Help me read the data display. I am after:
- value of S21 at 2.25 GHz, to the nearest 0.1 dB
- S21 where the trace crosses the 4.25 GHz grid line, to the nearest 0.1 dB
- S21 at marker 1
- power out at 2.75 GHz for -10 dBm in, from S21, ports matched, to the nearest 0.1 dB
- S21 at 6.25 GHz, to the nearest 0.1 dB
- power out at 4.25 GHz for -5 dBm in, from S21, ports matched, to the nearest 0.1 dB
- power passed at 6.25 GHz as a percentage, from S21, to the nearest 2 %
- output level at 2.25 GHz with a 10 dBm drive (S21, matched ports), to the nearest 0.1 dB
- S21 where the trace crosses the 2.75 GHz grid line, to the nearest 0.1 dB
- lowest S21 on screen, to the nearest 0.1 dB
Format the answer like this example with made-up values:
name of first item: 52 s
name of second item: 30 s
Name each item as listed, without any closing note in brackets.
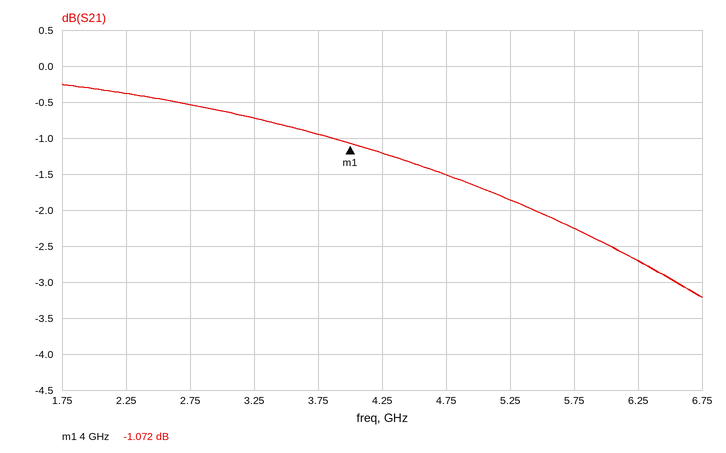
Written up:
value of S21 at 2.25 GHz, to the nearest 0.1 dB: -0.4 dB
S21 where the trace crosses the 4.25 GHz grid line, to the nearest 0.1 dB: -1.2 dB
S21 at marker 1: -1.072 dB
power out at 2.75 GHz for -10 dBm in, from S21, ports matched, to the nearest 0.1 dB: -10.5 dBm
S21 at 6.25 GHz, to the nearest 0.1 dB: -2.7 dB
power out at 4.25 GHz for -5 dBm in, from S21, ports matched, to the nearest 0.1 dB: -6.2 dBm
power passed at 6.25 GHz as a percentage, from S21, to the nearest 2 %: 54 %
output level at 2.25 GHz with a 10 dBm drive (S21, matched ports), to the nearest 0.1 dB: 9.6 dBm
S21 where the trace crosses the 2.75 GHz grid line, to the nearest 0.1 dB: -0.5 dB
lowest S21 on screen, to the nearest 0.1 dB: -3.2 dB
